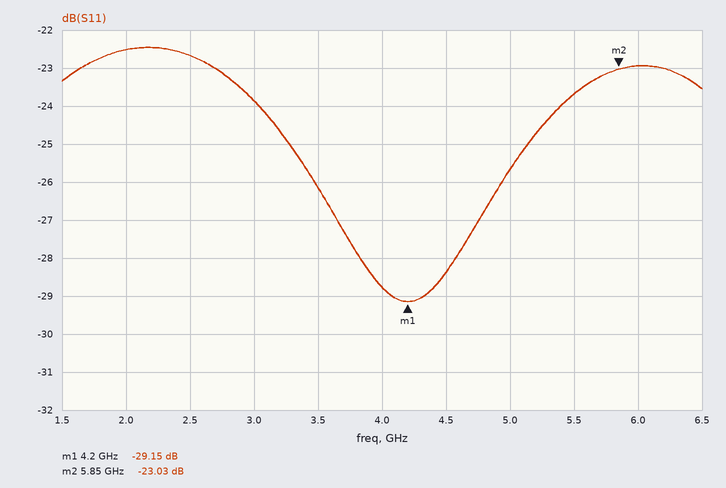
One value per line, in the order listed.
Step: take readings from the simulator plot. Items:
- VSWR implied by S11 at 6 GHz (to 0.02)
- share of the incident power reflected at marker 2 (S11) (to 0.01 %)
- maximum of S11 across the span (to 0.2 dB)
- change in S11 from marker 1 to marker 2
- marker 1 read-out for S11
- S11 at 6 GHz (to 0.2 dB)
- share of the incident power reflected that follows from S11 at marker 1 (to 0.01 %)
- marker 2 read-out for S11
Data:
1.16
0.50 %
-22.4 dB
6.12 dB
-29.15 dB
-23.0 dB
0.12 %
-23.03 dB
